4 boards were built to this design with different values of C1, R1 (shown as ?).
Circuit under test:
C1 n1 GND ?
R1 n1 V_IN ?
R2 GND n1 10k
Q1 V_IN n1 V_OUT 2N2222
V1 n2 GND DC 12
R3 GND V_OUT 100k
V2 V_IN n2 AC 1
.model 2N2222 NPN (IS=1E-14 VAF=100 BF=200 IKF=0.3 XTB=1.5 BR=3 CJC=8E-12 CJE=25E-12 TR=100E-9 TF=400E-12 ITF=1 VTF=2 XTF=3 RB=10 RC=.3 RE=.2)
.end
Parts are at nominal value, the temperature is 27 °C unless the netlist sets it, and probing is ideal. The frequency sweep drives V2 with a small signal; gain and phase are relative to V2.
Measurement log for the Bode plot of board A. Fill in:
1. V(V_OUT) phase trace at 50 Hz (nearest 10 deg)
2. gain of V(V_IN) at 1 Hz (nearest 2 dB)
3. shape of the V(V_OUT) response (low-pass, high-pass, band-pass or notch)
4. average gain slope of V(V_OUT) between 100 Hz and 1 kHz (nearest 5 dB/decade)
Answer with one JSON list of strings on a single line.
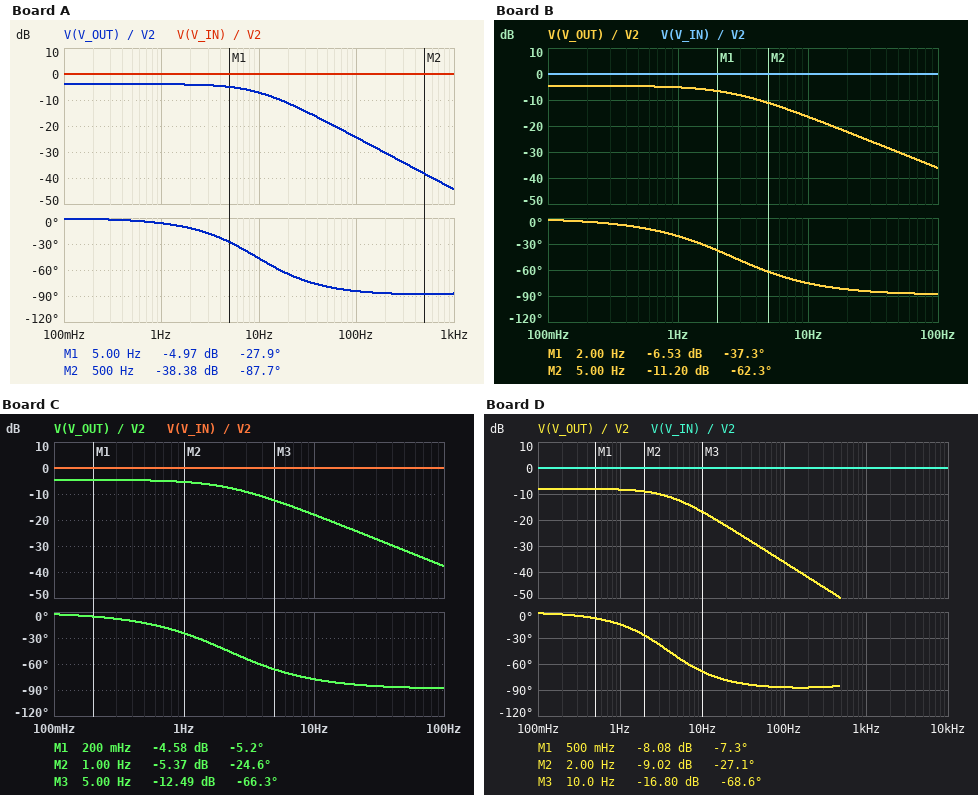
["-80 deg", "0 dB", "low-pass", "-20 dB/decade"]
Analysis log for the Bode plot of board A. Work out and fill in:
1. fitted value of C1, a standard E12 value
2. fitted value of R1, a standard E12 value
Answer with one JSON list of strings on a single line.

["4.7 µF", "5.6 kΩ"]
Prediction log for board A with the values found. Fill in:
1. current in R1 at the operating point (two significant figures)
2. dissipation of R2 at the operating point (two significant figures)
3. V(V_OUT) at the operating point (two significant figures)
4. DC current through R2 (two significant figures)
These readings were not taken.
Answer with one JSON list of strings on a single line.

["770 µA", "5.9 mW", "7.1 V", "770 µA"]
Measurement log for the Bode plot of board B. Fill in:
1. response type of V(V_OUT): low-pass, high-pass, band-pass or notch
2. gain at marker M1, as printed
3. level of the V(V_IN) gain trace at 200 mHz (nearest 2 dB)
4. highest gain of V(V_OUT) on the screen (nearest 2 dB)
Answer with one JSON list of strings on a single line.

["low-pass", "-6.53 dB", "0 dB", "-4 dB"]
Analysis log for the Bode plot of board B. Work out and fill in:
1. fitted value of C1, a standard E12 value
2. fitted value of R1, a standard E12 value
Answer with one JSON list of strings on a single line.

["15 µF", "6.8 kΩ"]
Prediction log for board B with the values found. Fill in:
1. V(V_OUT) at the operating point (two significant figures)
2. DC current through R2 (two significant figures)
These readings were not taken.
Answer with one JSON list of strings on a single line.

["6.6 V", "710 µA"]
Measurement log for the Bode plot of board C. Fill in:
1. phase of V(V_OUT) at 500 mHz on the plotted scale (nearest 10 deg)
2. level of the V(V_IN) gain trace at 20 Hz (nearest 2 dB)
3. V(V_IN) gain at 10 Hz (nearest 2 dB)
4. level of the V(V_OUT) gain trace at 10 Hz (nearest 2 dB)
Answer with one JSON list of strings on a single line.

["-10 deg", "0 dB", "0 dB", "-18 dB"]
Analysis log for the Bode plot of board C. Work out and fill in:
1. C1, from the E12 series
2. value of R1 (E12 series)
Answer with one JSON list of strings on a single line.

["18 µF", "6.8 kΩ"]
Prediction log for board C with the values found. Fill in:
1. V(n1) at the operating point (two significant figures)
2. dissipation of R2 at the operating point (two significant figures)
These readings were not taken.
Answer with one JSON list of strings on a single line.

["7.1 V", "5.1 mW"]
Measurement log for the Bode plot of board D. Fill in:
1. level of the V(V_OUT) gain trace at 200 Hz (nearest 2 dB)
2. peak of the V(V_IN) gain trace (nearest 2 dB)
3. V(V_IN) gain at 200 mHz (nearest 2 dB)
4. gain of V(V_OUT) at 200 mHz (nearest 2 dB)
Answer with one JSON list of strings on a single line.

["-42 dB", "0 dB", "0 dB", "-8 dB"]
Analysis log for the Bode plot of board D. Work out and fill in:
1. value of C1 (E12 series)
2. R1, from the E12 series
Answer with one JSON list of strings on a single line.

["6.8 µF", "15 kΩ"]
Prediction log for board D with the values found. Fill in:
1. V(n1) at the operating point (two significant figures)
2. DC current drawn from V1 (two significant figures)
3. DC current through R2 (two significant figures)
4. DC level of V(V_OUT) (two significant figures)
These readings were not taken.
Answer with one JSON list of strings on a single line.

["4.8 V", "520 µA", "480 µA", "4.2 V"]
